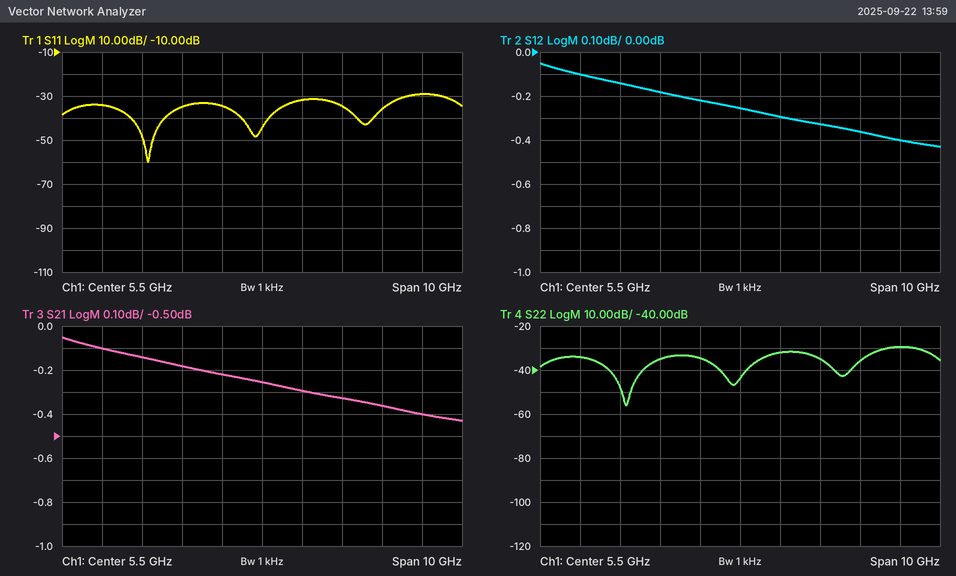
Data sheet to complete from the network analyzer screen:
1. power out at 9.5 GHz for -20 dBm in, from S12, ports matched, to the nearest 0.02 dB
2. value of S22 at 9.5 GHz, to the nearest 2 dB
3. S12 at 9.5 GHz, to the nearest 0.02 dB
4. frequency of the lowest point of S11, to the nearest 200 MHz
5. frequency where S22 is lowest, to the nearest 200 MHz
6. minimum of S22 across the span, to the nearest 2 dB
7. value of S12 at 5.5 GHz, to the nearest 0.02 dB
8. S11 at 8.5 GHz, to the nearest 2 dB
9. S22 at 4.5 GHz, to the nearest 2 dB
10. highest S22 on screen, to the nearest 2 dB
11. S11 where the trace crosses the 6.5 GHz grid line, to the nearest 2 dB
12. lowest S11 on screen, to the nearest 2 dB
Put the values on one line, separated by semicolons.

-20.40 dBm; -30 dB; -0.40 dB; 2.6 GHz; 2.6 GHz; -56 dB; -0.26 dB; -36 dB; -34 dB; -30 dB; -32 dB; -60 dB
